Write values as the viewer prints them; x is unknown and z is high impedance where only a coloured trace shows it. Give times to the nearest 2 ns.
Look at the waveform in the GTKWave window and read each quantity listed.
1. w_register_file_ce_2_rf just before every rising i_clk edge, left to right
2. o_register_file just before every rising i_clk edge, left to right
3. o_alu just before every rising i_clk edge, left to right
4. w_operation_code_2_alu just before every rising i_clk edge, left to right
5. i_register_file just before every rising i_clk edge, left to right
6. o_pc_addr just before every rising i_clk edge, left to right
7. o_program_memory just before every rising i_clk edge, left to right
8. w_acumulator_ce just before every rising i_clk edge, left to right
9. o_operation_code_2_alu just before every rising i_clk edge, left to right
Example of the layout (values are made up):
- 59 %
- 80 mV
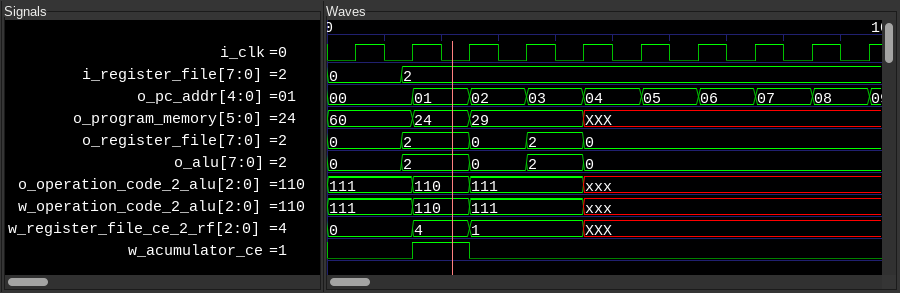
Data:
- 0, 0, 4, 1, 1, XXX, XXX, XXX, XXX, XXX
- 0, 2, 2, 0, 2, 0, 0, 0, 0, 0
- 0, 2, 2, 0, 2, 0, 0, 0, 0, 0
- 111, 111, 110, 111, 111, xxx, xxx, xxx, xxx, xxx
- 0, 2, 2, 2, 2, 2, 2, 2, 2, 2
- 00, 00, 01, 02, 03, 04, 05, 06, 07, 08
- 60, 60, 24, 29, 29, XXX, XXX, XXX, XXX, XXX
- 0 0 1 0 0 0 0 0 0 0
- 111, 111, 110, 111, 111, xxx, xxx, xxx, xxx, xxx
